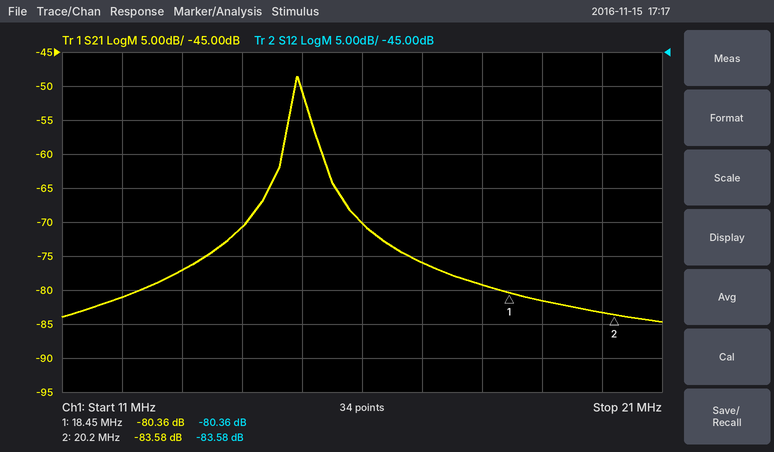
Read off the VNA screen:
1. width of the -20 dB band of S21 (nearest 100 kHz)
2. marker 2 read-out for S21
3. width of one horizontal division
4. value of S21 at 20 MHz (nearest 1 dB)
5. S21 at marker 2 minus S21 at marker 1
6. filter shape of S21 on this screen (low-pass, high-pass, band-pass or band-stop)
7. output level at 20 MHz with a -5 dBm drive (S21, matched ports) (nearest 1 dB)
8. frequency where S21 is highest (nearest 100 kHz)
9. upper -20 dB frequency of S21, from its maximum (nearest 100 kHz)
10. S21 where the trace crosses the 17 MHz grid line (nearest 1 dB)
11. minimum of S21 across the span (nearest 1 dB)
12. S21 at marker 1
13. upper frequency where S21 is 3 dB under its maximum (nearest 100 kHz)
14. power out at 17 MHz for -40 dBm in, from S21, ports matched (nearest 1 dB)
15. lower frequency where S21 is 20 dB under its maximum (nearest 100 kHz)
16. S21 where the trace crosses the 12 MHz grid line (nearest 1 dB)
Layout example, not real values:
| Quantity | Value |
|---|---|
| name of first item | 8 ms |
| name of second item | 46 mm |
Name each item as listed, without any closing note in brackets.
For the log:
| Quantity | Value |
|---|---|
| width of the -20 dB band of S21 | 1.6 MHz |
| marker 2 read-out for S21 | -83.58 dB |
| width of one horizontal division | 1 MHz |
| value of S21 at 20 MHz | -83 dB |
| S21 at marker 2 minus S21 at marker 1 | -3.22 dB |
| filter shape of S21 on this screen | band-pass |
| output level at 20 MHz with a -5 dBm drive (S21, matched ports) | -88 dBm |
| frequency where S21 is highest | 14.9 MHz |
| upper -20 dB frequency of S21, from its maximum | 15.8 MHz |
| S21 where the trace crosses the 17 MHz grid line | -76 dB |
| minimum of S21 across the span | -85 dB |
| S21 at marker 1 | -80.36 dB |
| upper frequency where S21 is 3 dB under its maximum | 15.0 MHz |
| power out at 17 MHz for -40 dBm in, from S21, ports matched | -116 dBm |
| lower frequency where S21 is 20 dB under its maximum | 14.2 MHz |
| S21 where the trace crosses the 12 MHz grid line | -81 dB |
